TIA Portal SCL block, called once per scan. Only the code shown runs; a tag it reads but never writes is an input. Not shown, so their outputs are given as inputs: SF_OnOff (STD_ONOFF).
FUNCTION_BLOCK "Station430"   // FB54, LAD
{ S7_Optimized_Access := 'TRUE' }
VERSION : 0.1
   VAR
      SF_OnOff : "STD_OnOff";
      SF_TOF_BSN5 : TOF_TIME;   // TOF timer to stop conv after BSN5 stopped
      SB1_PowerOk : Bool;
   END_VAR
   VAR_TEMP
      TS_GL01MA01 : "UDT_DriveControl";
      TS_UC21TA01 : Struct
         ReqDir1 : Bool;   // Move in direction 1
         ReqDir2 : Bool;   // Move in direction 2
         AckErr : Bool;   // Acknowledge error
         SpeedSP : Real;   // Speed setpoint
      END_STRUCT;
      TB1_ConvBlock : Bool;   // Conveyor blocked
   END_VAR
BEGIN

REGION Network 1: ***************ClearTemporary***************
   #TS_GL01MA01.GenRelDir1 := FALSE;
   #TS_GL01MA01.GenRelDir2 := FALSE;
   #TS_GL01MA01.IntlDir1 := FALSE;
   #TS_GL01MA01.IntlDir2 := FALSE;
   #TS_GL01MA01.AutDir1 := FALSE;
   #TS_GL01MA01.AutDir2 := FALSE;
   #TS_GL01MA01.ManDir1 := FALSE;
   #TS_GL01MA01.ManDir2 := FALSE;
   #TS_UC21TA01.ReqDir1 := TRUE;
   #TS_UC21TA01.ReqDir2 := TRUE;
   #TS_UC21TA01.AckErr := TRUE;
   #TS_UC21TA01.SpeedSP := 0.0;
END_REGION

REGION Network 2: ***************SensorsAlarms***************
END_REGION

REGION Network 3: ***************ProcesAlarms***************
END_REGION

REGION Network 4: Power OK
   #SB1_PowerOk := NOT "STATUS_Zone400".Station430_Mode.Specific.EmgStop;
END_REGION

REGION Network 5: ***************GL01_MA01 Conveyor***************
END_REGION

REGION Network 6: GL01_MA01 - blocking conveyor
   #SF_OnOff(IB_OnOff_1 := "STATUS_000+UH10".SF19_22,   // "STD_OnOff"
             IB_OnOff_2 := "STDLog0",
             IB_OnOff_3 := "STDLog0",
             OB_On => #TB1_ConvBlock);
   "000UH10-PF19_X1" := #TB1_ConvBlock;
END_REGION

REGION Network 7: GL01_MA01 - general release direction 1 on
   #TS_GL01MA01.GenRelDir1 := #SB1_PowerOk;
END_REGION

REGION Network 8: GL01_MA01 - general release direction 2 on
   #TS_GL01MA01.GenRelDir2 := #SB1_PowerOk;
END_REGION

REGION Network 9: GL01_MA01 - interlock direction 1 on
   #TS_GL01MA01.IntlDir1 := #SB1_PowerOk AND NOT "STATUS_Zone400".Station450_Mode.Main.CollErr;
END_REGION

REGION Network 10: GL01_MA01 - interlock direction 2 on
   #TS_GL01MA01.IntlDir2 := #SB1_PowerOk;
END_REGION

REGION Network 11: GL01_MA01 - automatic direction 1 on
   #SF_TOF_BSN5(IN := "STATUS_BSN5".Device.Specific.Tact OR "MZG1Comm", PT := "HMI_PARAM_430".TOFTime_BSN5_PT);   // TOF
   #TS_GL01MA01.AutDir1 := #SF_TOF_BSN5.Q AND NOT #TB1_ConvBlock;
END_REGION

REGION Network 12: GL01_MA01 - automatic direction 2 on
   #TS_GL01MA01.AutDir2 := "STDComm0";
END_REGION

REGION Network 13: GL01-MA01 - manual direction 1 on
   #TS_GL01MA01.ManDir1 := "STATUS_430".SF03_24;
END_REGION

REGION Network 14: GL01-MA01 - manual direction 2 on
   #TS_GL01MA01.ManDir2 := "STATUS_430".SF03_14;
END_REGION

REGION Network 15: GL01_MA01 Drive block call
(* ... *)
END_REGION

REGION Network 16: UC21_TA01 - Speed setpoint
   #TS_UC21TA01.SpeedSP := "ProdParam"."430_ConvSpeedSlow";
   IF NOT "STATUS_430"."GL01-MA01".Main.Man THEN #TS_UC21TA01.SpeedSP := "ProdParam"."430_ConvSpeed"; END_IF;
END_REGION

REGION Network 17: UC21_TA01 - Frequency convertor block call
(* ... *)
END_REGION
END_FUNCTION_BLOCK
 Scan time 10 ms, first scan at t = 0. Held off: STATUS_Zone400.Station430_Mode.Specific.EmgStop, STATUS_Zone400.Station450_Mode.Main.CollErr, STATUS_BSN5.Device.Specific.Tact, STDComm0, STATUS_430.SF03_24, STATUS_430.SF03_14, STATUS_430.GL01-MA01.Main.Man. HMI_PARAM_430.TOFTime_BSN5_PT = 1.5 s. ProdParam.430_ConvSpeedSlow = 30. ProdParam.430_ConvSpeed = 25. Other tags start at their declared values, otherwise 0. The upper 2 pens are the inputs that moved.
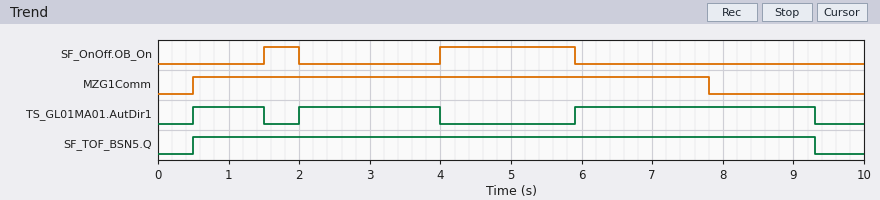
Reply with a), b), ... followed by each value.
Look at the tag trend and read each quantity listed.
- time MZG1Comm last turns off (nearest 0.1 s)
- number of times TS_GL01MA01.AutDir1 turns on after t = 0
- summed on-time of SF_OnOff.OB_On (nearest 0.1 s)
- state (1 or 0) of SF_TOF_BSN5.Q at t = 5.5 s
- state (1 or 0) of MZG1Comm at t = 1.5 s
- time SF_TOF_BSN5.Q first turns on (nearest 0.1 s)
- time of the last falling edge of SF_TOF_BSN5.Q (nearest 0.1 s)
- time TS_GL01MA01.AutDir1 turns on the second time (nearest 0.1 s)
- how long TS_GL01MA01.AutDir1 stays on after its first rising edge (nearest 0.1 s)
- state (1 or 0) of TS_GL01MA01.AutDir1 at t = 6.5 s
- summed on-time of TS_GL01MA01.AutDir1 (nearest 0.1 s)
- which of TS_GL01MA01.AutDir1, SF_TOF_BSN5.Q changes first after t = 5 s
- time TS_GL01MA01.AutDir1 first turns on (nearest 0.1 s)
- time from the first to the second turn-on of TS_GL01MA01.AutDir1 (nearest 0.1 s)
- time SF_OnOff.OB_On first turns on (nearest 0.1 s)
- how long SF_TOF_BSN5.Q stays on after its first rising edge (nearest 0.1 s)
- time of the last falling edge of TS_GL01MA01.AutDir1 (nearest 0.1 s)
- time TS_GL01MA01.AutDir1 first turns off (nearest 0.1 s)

a) 7.8 s
b) 3
c) 2.4 s
d) 1
e) 1
f) 0.5 s
g) 9.3 s
h) 2.0 s
i) 1.0 s
j) 1
k) 6.4 s
l) TS_GL01MA01.AutDir1
m) 0.5 s
n) 1.5 s
o) 1.5 s
p) 8.8 s
q) 9.3 s
r) 1.5 s
